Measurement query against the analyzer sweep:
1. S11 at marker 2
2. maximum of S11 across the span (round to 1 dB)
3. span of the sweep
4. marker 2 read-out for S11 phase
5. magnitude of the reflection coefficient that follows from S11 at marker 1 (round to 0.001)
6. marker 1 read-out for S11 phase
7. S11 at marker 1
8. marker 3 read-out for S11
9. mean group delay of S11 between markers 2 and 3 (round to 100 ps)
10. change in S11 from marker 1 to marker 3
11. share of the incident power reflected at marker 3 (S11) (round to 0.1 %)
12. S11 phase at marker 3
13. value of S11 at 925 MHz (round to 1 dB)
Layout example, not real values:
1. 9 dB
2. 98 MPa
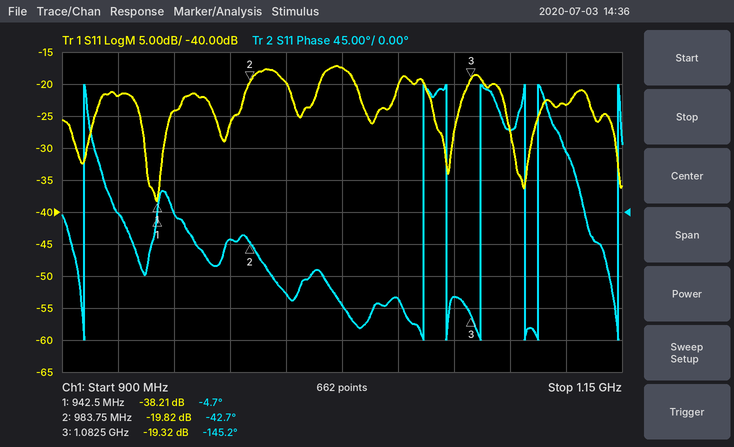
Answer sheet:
1. -19.82 dB
2. -17 dB
3. 250 MHz
4. -42.7°
5. 0.012
6. -4.7°
7. -38.21 dB
8. -19.32 dB
9. 2.9 ns
10. 18.89 dB
11. 1.2 %
12. -145.2°
13. -22 dB
